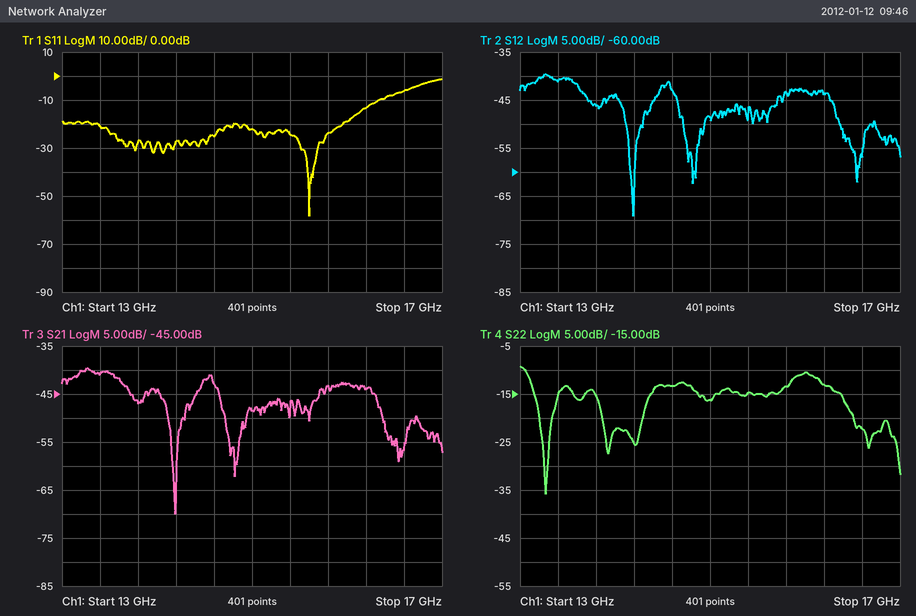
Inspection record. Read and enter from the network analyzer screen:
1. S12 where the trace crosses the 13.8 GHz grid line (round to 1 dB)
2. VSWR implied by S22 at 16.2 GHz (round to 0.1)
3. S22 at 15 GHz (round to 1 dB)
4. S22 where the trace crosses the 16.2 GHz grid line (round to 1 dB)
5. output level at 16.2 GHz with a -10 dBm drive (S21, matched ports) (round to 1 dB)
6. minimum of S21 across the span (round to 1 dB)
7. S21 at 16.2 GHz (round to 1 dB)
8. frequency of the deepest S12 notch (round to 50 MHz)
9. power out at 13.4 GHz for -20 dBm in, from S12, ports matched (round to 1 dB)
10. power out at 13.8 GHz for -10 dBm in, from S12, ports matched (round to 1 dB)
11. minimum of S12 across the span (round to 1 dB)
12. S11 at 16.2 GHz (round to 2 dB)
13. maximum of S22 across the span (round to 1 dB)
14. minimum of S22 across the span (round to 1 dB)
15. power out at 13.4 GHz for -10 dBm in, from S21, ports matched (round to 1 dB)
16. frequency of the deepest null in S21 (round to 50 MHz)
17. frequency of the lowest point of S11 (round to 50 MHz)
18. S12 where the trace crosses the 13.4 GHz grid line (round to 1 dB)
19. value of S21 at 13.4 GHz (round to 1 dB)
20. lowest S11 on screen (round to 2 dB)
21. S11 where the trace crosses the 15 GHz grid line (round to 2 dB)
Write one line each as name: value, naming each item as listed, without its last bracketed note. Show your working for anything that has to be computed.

S12 where the trace crosses the 13.8 GHz grid line: -46 dB
VSWR implied by S22 at 16.2 GHz: |Γ| = 10^(-13/20) = 0.2239; VSWR = (1 + 0.2239)/(1 − 0.2239) ≈ 1.6
S22 at 15 GHz: -16 dB
S22 where the trace crosses the 16.2 GHz grid line: -13 dB
output level at 16.2 GHz with a -10 dBm drive (S21, matched ports): -10 dBm + (-44 dB) = -54 dBm
minimum of S21 across the span: -70 dB
S21 at 16.2 GHz: -44 dB
frequency of the deepest S12 notch: 14.20 GHz
power out at 13.4 GHz for -20 dBm in, from S12, ports matched: -20 dBm + (-41 dB) = -61 dBm
power out at 13.8 GHz for -10 dBm in, from S12, ports matched: -10 dBm + (-46 dB) = -56 dBm
minimum of S12 across the span: -69 dB
S11 at 16.2 GHz: -14 dB
maximum of S22 across the span: -9 dB
minimum of S22 across the span: -36 dB
power out at 13.4 GHz for -10 dBm in, from S21, ports matched: -10 dBm + (-41 dB) = -51 dBm
frequency of the deepest null in S21: 14.20 GHz
frequency of the lowest point of S11: 15.60 GHz
S12 where the trace crosses the 13.4 GHz grid line: -41 dB
value of S21 at 13.4 GHz: -41 dB
lowest S11 on screen: -58 dB
S11 where the trace crosses the 15 GHz grid line: -22 dB
